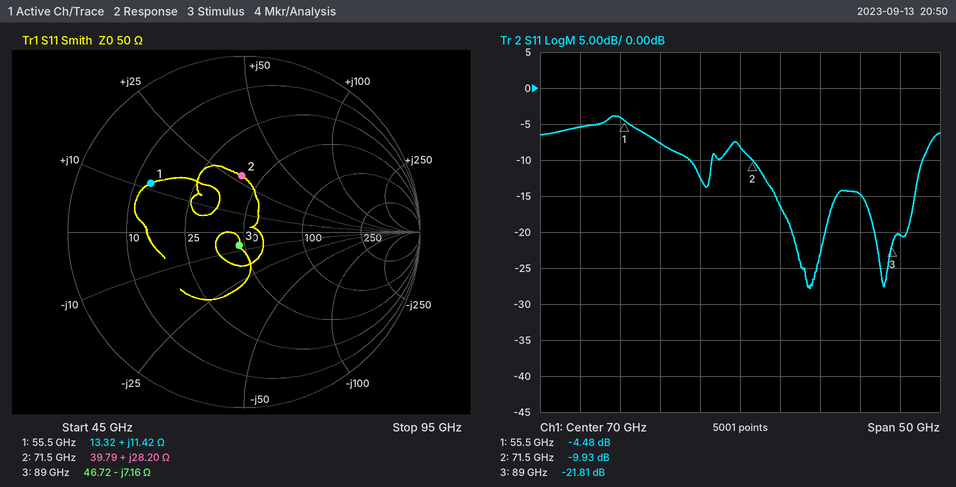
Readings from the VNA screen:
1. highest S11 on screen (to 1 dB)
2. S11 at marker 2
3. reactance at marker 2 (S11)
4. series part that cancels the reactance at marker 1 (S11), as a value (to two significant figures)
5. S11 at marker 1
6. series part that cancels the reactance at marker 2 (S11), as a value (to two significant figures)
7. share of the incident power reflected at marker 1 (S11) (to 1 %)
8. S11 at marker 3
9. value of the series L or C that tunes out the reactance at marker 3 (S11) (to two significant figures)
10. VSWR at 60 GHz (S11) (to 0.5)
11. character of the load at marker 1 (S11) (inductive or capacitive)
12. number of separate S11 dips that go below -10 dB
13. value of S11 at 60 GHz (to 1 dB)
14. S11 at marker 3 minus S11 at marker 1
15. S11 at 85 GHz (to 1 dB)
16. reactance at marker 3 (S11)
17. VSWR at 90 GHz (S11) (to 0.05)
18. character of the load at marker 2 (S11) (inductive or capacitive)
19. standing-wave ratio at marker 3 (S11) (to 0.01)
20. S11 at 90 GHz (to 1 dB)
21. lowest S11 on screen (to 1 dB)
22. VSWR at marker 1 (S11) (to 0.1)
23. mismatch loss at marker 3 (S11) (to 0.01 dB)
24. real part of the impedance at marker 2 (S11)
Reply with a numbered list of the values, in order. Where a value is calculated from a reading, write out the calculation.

1. -4 dB
2. -9.93 dB
3. +28.20 Ω
4. C = 1/(2π × 55.5 GHz × 11.42 Ω) ≈ 251 fF, so 250 fF to two significant figures
5. -4.48 dB
6. C = 1/(2π × 71.5 GHz × 28.2 Ω) ≈ 79 fF
7. 10^(-4.48/10) ≈ 36 %
8. -21.81 dB
9. L = 7.16 Ω/(2π × 89 GHz) ≈ 13 pH
10. |Γ| = 10^(-8/20) = 0.3981; VSWR = (1 + 0.3981)/(1 − 0.3981) ≈ 2.32, so 2.5 to the nearest 0.5
11. inductive
12. 3
13. -8 dB
14. -21.81 − (-4.48) = -17.33 dB
15. -15 dB
16. -7.16 Ω
17. |Γ| = 10^(-20/20) = 0.1000; VSWR = (1 + 0.1000)/(1 − 0.1000) ≈ 1.22, so 1.20 to the nearest 0.05
18. inductive
19. 1.18
20. -20 dB
21. -28 dB
22. 4.0
23. −10 log10(1 − 10^(-21.81/10)) ≈ 0.03 dB
24. 39.79 Ω
